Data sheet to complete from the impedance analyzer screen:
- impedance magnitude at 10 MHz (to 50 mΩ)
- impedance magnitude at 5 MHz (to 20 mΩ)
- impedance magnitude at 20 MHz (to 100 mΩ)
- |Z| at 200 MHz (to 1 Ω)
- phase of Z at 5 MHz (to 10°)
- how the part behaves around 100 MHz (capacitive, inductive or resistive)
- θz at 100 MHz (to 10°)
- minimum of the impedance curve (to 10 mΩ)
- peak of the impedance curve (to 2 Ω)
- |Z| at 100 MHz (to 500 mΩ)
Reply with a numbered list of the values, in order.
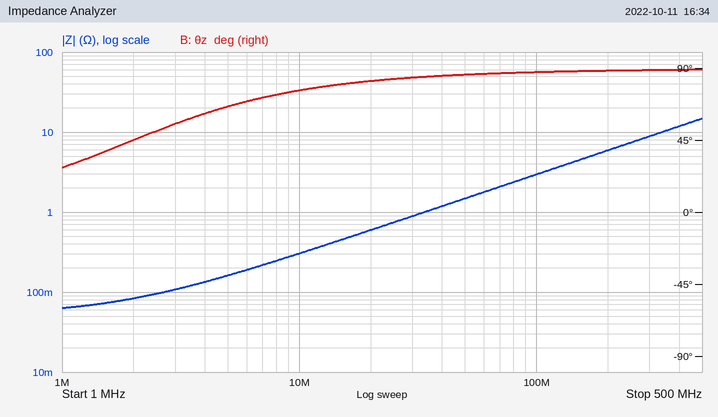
1. 300 mΩ
2. 160 mΩ
3. 600 mΩ
4. 6 Ω
5. 70°
6. inductive
7. 90°
8. 60 mΩ
9. 14 Ω
10. 3.0 Ω
